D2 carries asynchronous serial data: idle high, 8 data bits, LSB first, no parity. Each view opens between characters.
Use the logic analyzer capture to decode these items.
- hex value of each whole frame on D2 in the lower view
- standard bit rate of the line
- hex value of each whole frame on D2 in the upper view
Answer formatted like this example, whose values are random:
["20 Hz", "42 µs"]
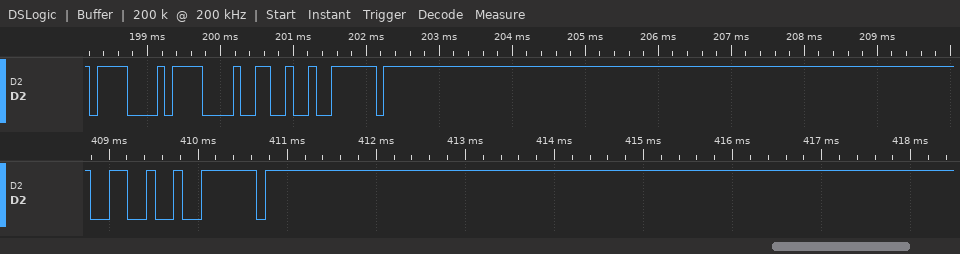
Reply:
["26, 7E", "9600 baud", "0F, 0F, 26, 7E"]
